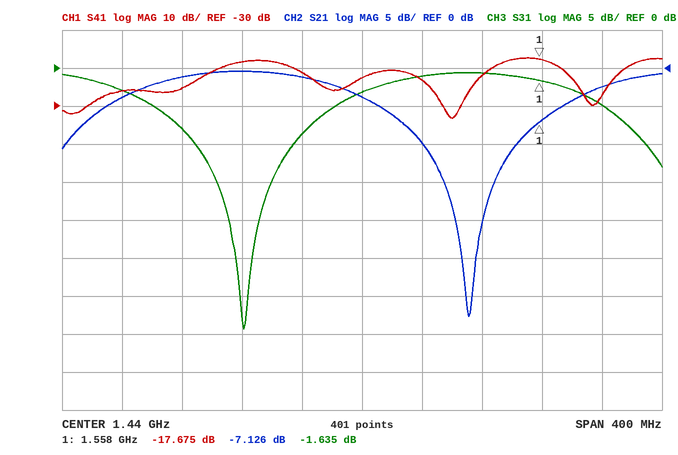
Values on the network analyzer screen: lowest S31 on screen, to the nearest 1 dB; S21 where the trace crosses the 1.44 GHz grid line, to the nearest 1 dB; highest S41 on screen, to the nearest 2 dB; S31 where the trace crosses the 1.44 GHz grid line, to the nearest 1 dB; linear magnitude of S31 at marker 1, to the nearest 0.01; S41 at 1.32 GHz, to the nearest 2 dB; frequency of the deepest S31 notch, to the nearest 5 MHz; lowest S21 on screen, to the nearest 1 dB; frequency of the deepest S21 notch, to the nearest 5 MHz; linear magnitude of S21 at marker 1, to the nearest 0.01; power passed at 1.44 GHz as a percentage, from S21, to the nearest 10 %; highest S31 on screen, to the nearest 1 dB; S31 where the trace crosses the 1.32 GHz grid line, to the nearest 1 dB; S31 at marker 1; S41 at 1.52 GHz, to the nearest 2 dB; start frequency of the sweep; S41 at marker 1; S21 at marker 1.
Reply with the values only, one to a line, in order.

-34 dB
-4 dB
-18 dB
-3 dB
0.83
-26 dB
1.360 GHz
-33 dB
1.510 GHz
0.44
40 %
-1 dB
-8 dB
-1.635 dB
-22 dB
1.24 GHz
-17.675 dB
-7.126 dB
